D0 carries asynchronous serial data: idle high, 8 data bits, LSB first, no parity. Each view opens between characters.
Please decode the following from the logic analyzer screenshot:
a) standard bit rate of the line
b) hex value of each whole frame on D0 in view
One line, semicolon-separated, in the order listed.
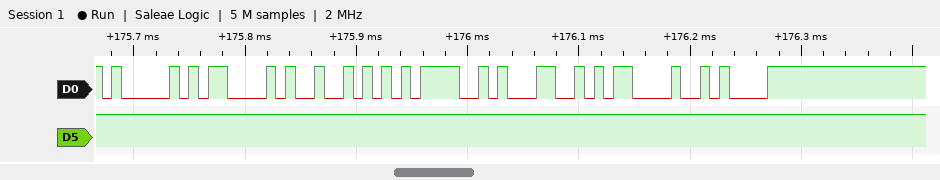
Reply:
115200 baud; 41, 43, 52, 3D, 31, 0D, 0A
